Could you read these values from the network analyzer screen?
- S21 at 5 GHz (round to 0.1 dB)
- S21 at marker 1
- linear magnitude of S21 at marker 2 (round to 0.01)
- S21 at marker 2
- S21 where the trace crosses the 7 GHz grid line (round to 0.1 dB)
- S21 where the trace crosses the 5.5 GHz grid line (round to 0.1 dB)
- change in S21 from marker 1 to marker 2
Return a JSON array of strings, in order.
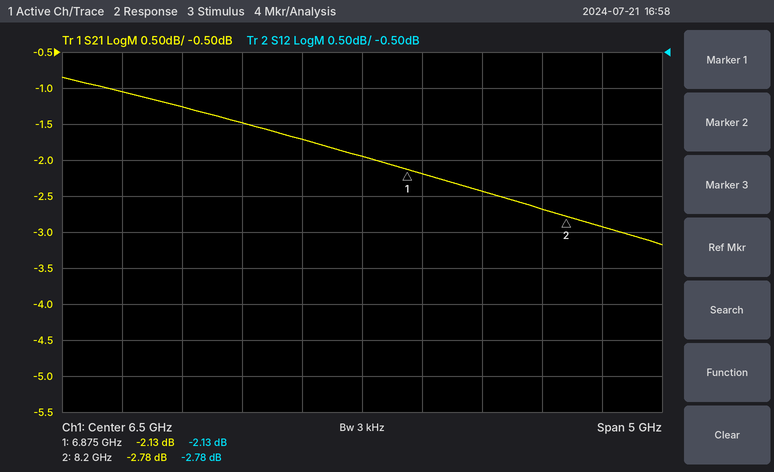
["-1.3 dB", "-2.13 dB", "0.73", "-2.78 dB", "-2.2 dB", "-1.5 dB", "-0.65 dB"]
